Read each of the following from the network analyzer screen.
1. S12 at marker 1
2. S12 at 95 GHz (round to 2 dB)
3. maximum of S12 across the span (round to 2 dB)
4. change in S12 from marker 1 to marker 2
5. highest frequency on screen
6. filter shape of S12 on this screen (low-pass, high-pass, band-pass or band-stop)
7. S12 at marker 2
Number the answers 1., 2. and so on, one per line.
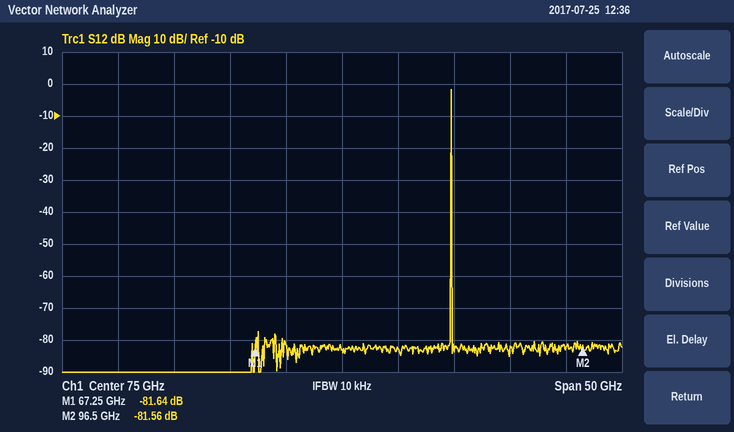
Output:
1. -81.64 dB
2. -82 dB
3. -2 dB
4. 0.08 dB
5. 100 GHz
6. band-pass
7. -81.56 dB
